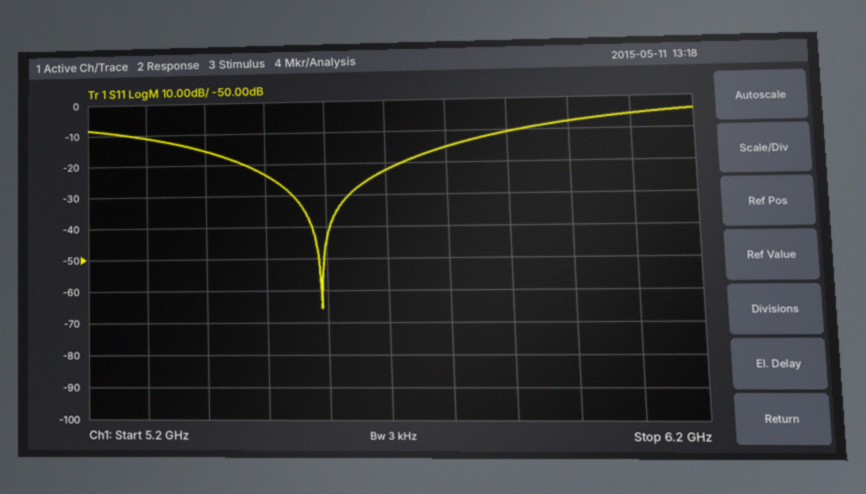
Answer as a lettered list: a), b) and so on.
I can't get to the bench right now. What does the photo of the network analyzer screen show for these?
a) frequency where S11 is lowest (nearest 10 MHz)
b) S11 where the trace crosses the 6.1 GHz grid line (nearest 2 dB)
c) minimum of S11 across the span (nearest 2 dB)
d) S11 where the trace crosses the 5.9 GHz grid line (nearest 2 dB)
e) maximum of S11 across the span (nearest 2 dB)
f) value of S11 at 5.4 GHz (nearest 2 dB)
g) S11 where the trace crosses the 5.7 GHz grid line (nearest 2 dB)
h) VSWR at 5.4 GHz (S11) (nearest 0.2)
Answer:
a) 5.59 GHz
b) -6 dB
c) -66 dB
d) -10 dB
e) -4 dB
f) -16 dB
g) -22 dB
h) 1.4
